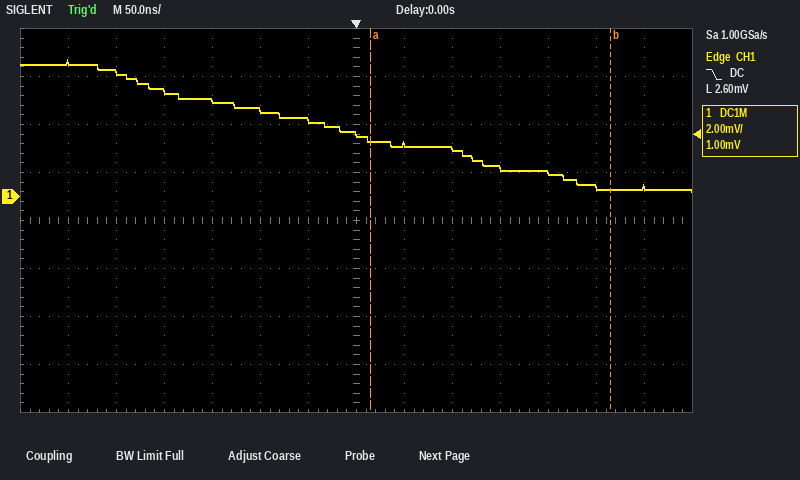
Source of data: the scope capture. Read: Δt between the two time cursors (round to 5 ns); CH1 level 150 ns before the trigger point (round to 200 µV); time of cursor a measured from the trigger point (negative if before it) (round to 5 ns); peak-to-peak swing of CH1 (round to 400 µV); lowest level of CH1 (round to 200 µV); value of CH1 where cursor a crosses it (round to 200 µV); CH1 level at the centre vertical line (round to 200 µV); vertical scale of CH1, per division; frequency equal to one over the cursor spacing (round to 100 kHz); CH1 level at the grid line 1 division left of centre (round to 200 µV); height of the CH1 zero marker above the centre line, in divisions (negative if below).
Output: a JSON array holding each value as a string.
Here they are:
["250 ns", "4.0 mV", "+15 ns", "5.6 mV", "200 µV", "2.4 mV", "2.6 mV", "2 mV", "4.0 MHz", "3.2 mV", "+0.5 div"]
